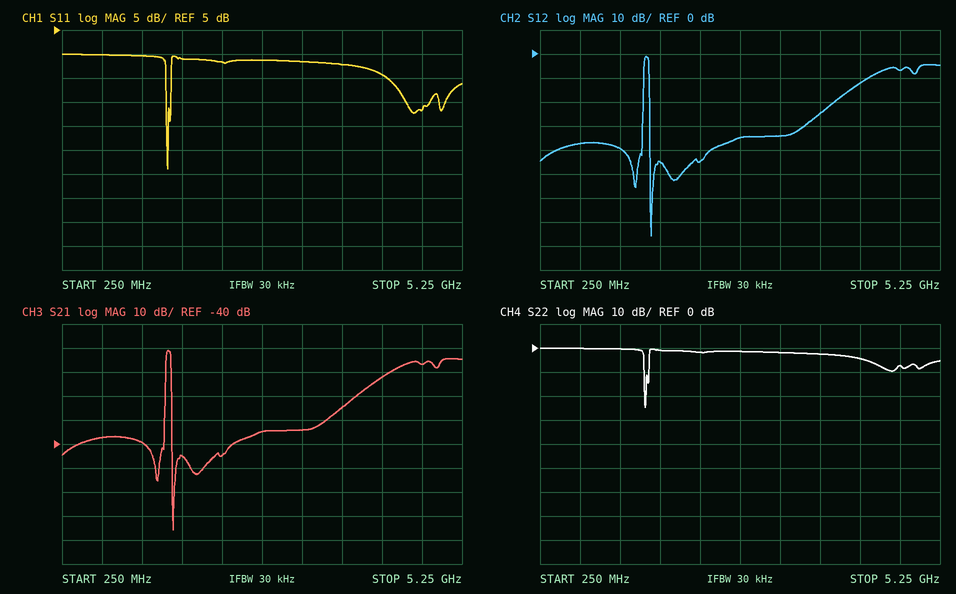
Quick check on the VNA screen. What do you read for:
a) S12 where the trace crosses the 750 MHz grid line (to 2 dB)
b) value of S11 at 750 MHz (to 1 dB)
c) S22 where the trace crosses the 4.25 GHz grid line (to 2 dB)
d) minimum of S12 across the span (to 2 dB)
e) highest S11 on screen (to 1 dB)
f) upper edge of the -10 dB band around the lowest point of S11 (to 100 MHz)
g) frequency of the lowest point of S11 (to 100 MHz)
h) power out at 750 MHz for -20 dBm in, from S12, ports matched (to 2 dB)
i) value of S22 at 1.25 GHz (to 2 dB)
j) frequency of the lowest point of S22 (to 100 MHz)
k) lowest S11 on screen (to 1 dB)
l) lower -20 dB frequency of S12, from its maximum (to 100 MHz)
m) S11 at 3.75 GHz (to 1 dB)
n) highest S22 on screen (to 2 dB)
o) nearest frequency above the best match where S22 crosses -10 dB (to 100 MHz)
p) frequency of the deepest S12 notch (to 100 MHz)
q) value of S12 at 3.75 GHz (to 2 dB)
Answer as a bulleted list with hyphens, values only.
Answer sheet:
- -38 dB
- 0 dB
- -4 dB
- -76 dB
- 0 dB
- 1.6 GHz
- 1.6 GHz
- -58 dBm
- 0 dB
- 1.6 GHz
- -24 dB
- 1.5 GHz
- -2 dB
- 0 dB
- 1.6 GHz
- 1.6 GHz
- -24 dB
